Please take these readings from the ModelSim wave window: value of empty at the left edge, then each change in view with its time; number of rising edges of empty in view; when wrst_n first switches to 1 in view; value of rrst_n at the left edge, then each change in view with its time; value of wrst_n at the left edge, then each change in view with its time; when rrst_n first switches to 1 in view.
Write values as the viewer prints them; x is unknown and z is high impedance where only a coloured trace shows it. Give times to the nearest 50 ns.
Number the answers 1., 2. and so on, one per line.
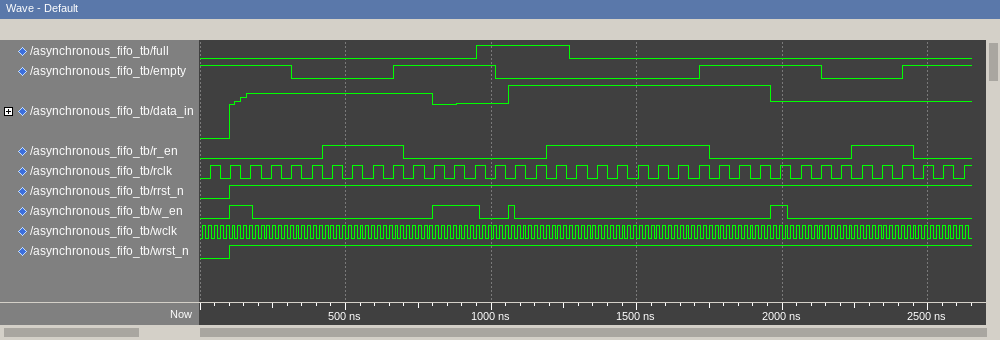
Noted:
1. 1, 0 at 300 ns, 1 at 650 ns, 0 at 1000 ns, 1 at 1700 ns, 0 at 2150 ns, 1 at 2400 ns
2. 3
3. 100 ns
4. 0, 1 at 100 ns
5. 0, 1 at 100 ns
6. 100 ns
